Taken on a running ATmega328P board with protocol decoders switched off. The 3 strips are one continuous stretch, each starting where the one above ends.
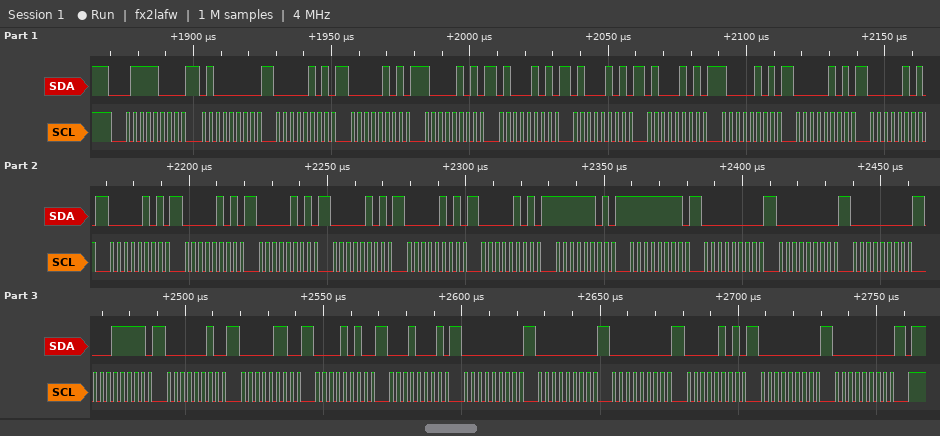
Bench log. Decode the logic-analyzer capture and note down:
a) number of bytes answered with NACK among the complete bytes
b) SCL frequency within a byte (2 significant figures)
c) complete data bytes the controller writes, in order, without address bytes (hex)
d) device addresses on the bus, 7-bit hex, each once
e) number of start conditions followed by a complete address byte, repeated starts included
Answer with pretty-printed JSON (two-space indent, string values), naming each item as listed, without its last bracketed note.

{
  "number of bytes answered with NACK among the complete bytes": "0",
  "SCL frequency within a byte": "400 kHz",
  "complete data bytes the controller writes, in order, without address bytes": "40 05 05 85 45 45 45 85 05 05 05 05 05 05 05 05 FD FF 00 00 00 1F 02 06 0A 11 00 00 00 05 00 00",
  "device addresses on the bus, 7-bit hex, each once": "0x3C",
  "number of start conditions followed by a complete address byte, repeated starts included": "1"
}
